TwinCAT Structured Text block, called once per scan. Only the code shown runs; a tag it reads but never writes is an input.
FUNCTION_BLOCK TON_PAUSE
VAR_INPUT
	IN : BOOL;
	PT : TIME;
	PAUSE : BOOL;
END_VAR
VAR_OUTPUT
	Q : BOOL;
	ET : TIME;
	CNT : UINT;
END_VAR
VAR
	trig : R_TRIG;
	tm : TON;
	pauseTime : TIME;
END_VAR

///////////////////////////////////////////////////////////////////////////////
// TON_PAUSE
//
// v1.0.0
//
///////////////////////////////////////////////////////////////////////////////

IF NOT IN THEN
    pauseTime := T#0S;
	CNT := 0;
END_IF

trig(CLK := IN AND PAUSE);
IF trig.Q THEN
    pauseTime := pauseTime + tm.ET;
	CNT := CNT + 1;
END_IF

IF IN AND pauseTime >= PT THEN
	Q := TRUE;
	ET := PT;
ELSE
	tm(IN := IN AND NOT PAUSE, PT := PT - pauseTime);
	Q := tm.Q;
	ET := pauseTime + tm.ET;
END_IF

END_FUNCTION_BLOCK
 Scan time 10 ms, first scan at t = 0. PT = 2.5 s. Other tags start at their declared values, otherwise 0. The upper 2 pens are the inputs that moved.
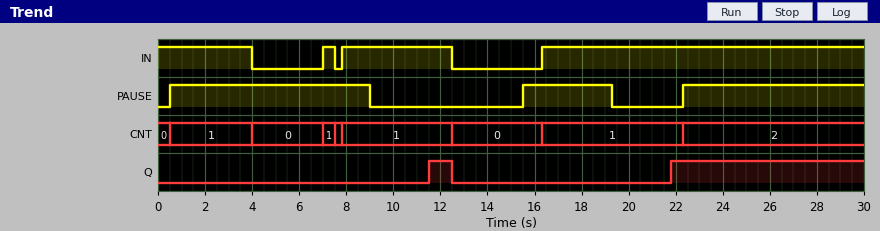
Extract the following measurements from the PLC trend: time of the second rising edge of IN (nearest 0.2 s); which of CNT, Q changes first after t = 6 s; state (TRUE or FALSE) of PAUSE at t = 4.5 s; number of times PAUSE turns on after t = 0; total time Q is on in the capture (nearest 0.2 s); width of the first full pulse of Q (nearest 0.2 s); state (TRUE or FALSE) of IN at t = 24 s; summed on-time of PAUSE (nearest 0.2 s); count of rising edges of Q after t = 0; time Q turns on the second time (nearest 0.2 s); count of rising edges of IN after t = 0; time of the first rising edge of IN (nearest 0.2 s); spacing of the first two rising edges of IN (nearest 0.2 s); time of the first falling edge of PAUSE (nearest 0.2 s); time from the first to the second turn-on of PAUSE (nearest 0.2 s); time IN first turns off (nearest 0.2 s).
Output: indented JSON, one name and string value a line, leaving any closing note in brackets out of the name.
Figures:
{
  "time of the second rising edge of IN": "7.8 s",
  "which of CNT, Q changes first after t = 6 s": "CNT",
  "state (TRUE or FALSE) of PAUSE at t = 4.5 s": "TRUE",
  "number of times PAUSE turns on after t = 0": "3",
  "total time Q is on in the capture": "9.2 s",
  "width of the first full pulse of Q": "1.0 s",
  "state (TRUE or FALSE) of IN at t = 24 s": "TRUE",
  "summed on-time of PAUSE": "20.0 s",
  "count of rising edges of Q after t = 0": "2",
  "time Q turns on the second time": "21.8 s",
  "count of rising edges of IN after t = 0": "3",
  "time of the first rising edge of IN": "7.0 s",
  "spacing of the first two rising edges of IN": "0.8 s",
  "time of the first falling edge of PAUSE": "9.0 s",
  "time from the first to the second turn-on of PAUSE": "15.0 s",
  "time IN first turns off": "4.0 s"
}
